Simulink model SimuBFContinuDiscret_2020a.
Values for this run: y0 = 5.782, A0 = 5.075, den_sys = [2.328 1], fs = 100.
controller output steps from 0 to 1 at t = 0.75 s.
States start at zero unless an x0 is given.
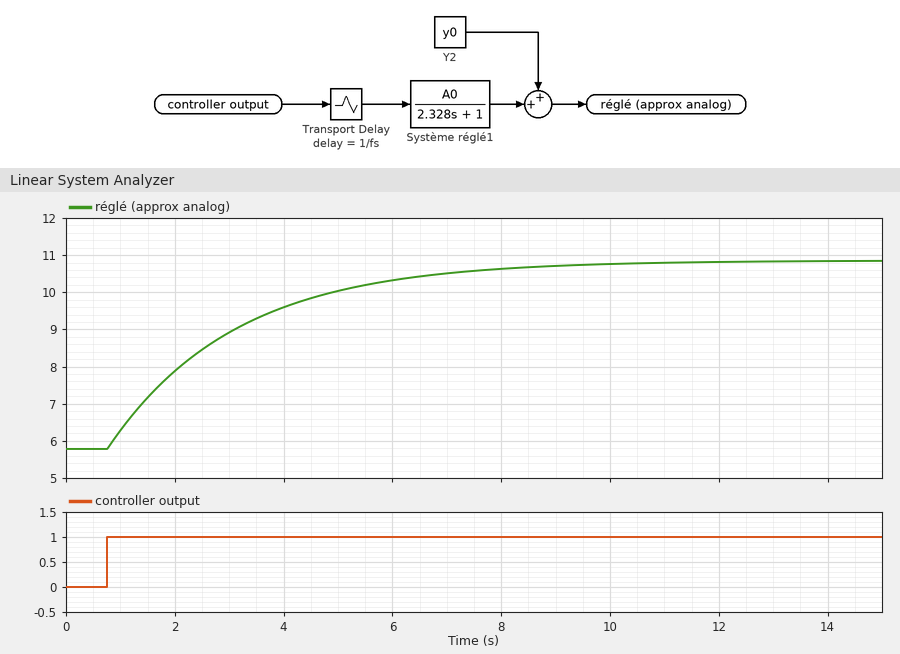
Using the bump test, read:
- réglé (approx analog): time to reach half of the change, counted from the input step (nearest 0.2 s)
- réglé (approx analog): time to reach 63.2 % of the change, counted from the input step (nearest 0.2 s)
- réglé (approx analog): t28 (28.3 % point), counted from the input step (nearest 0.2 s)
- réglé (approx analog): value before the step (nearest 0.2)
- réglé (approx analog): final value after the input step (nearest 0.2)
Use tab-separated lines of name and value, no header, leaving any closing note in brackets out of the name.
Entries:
réglé (approx analog): time to reach half of the change, counted from the input step	1.6 s
réglé (approx analog): time to reach 63.2 % of the change, counted from the input step	2.4 s
réglé (approx analog): t28 (28.3 % point), counted from the input step	0.8 s
réglé (approx analog): value before the step	5.8
réglé (approx analog): final value after the input step	10.8
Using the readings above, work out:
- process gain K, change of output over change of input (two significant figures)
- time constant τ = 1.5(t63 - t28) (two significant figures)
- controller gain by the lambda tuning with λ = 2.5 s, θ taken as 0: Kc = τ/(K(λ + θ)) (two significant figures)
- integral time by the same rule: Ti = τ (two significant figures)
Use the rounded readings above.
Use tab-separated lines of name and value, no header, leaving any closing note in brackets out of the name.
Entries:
process gain K, change of output over change of input	5.0
time constant τ = 1.5(t63 - t28)	2.4 s
controller gain by the lambda tuning with λ = 2.5 s, θ taken as 0: Kc = τ/(K(λ + θ))	0.19
integral time by the same rule: Ti = τ	2.4 s
